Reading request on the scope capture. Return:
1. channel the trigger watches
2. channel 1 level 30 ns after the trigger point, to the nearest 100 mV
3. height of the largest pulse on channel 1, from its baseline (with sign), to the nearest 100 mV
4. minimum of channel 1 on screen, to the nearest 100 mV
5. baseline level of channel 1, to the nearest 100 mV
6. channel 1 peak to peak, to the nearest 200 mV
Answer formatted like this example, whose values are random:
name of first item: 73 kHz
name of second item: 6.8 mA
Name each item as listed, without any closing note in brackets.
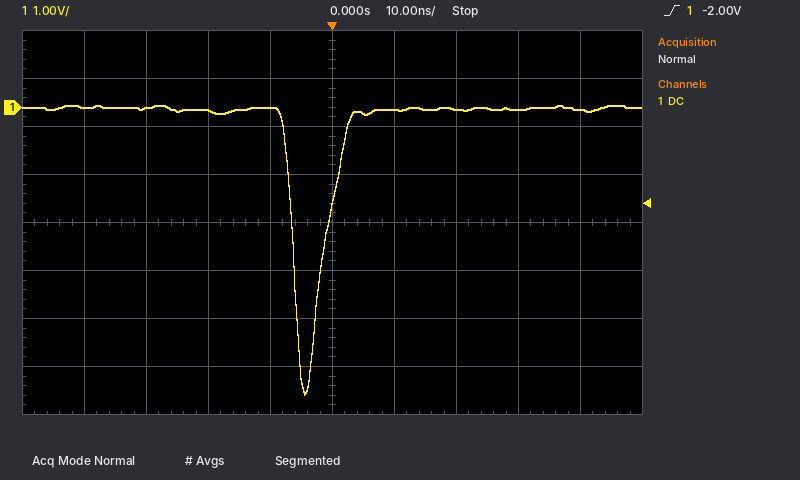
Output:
channel the trigger watches: channel 1
channel 1 level 30 ns after the trigger point, to the nearest 100 mV: 0.0 V
height of the largest pulse on channel 1, from its baseline (with sign), to the nearest 100 mV: -6.0 V
minimum of channel 1 on screen, to the nearest 100 mV: -6.0 V
baseline level of channel 1, to the nearest 100 mV: 0.0 V
channel 1 peak to peak, to the nearest 200 mV: 6.0 V
